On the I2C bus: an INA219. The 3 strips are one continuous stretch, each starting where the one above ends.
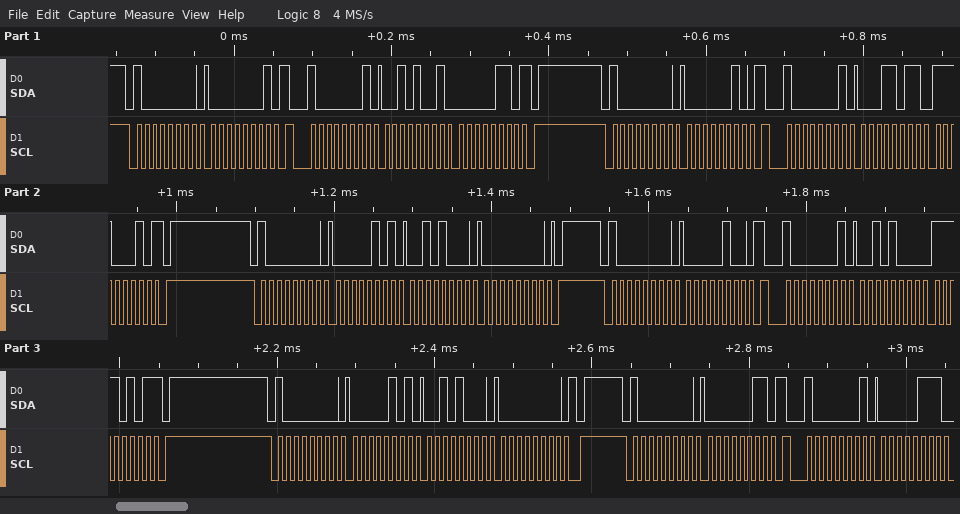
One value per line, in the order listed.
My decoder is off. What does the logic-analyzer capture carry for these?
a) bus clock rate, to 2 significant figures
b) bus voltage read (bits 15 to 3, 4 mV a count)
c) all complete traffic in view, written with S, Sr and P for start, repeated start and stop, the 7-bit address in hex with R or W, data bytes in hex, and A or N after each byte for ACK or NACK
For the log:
100 kHz
3.568 V
S 40W A 01 A Sr 40R A 29 A 06 N P S 40W A 02 A Sr 40R A 1B A E2 N P S 40W A 05 A 28 A 00 A P S 40W A 04 A Sr 40R A 28 A F5 N P S 40W A 05 A 28 A 00 A P S 40W A 03 A Sr 40R A 07 A
